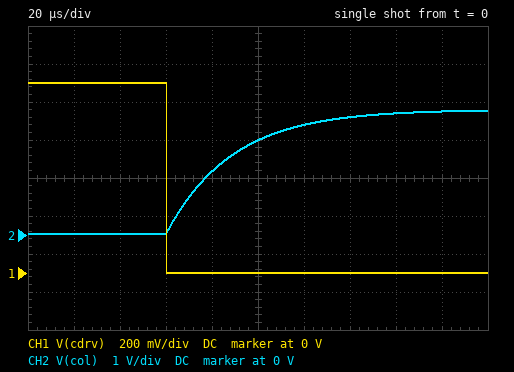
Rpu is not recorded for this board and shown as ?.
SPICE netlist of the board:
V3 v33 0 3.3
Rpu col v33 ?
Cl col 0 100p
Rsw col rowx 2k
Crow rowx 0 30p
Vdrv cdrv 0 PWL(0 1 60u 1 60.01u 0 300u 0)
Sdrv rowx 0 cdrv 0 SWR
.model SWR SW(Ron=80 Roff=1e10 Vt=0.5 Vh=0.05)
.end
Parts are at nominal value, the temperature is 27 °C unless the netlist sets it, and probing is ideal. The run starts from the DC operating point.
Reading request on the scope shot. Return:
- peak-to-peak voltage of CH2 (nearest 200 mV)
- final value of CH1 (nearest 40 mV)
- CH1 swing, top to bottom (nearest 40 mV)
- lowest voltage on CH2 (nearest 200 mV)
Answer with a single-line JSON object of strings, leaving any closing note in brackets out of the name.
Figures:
{"peak-to-peak voltage of CH2": "3.2 V", "final value of CH1": "0 V", "CH1 swing, top to bottom": "1.00 V", "lowest voltage on CH2": "0 V"}
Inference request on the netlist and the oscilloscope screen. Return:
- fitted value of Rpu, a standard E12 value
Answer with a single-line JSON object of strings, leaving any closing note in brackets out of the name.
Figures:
{"fitted value of Rpu, a standard E12 value": "220 kΩ"}
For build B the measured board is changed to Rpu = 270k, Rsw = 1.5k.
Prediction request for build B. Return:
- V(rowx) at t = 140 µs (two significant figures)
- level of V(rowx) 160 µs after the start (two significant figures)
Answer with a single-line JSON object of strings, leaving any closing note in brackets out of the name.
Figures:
{"V(rowx) at t = 140 µs": "3.0 V", "level of V(rowx) 160 µs after the start": "3.1 V"}
